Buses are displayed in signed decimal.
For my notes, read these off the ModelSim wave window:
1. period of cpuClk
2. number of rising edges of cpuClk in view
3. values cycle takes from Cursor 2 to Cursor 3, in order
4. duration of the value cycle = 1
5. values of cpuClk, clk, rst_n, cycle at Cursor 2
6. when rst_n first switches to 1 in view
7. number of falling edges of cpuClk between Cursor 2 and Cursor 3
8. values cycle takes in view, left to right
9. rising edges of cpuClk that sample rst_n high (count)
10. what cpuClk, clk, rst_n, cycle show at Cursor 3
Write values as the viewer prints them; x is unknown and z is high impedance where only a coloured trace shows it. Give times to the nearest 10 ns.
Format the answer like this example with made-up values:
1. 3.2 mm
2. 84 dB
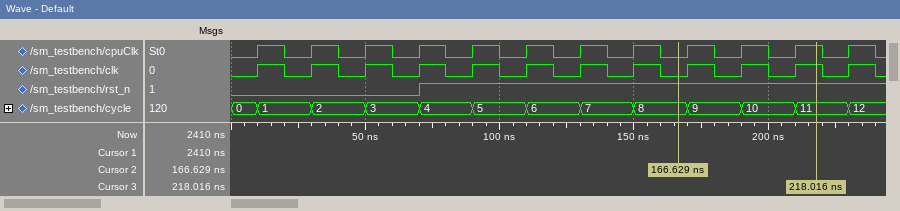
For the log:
1. 20 ns
2. 12
3. 8, 9, 10, 11
4. 20 ns
5. cpuClk=0, clk=0, rst_n=1, cycle=8
6. 70 ns
7. 2
8. 0, 1, 2, 3, 4, 5, 6, 7, 8, 9, 10, 11, 12
9. 8
10. cpuClk=1, clk=1, rst_n=1, cycle=11
